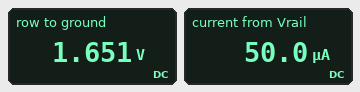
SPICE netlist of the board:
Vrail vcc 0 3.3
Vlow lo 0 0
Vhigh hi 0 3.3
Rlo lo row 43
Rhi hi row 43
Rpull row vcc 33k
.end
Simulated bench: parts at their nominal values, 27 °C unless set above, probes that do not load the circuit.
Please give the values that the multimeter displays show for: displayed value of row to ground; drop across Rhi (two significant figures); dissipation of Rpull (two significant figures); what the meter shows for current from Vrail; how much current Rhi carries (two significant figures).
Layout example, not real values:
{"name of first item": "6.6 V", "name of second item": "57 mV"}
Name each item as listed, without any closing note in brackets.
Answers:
{"displayed value of row to ground": "1.651 V", "drop across Rhi": "1.6 V", "dissipation of Rpull": "82 µW", "what the meter shows for current from Vrail": "50.0 µA", "how much current Rhi carries": "38 mA"}
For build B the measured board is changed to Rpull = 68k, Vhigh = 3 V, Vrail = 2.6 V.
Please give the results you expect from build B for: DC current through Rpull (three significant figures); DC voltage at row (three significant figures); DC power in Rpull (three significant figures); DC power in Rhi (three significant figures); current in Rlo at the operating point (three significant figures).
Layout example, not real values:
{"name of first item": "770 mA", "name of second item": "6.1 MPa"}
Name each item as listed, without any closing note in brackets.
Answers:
{"DC current through Rpull": "16.2 µA", "DC voltage at row": "1.50 V", "DC power in Rpull": "17.8 µW", "DC power in Rhi": "52.3 mW", "current in Rlo at the operating point": "34.9 mA"}
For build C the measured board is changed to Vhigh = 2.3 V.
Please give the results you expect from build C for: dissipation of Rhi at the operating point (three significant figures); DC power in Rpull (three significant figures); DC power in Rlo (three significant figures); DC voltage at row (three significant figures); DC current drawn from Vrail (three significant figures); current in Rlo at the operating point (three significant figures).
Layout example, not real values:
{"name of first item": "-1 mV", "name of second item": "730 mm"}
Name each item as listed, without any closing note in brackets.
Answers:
{"dissipation of Rhi at the operating point": "30.7 mW", "DC power in Rpull": "140 µW", "DC power in Rlo": "30.8 mW", "DC voltage at row": "1.15 V", "DC current drawn from Vrail": "65.1 µA", "current in Rlo at the operating point": "26.8 mA"}
